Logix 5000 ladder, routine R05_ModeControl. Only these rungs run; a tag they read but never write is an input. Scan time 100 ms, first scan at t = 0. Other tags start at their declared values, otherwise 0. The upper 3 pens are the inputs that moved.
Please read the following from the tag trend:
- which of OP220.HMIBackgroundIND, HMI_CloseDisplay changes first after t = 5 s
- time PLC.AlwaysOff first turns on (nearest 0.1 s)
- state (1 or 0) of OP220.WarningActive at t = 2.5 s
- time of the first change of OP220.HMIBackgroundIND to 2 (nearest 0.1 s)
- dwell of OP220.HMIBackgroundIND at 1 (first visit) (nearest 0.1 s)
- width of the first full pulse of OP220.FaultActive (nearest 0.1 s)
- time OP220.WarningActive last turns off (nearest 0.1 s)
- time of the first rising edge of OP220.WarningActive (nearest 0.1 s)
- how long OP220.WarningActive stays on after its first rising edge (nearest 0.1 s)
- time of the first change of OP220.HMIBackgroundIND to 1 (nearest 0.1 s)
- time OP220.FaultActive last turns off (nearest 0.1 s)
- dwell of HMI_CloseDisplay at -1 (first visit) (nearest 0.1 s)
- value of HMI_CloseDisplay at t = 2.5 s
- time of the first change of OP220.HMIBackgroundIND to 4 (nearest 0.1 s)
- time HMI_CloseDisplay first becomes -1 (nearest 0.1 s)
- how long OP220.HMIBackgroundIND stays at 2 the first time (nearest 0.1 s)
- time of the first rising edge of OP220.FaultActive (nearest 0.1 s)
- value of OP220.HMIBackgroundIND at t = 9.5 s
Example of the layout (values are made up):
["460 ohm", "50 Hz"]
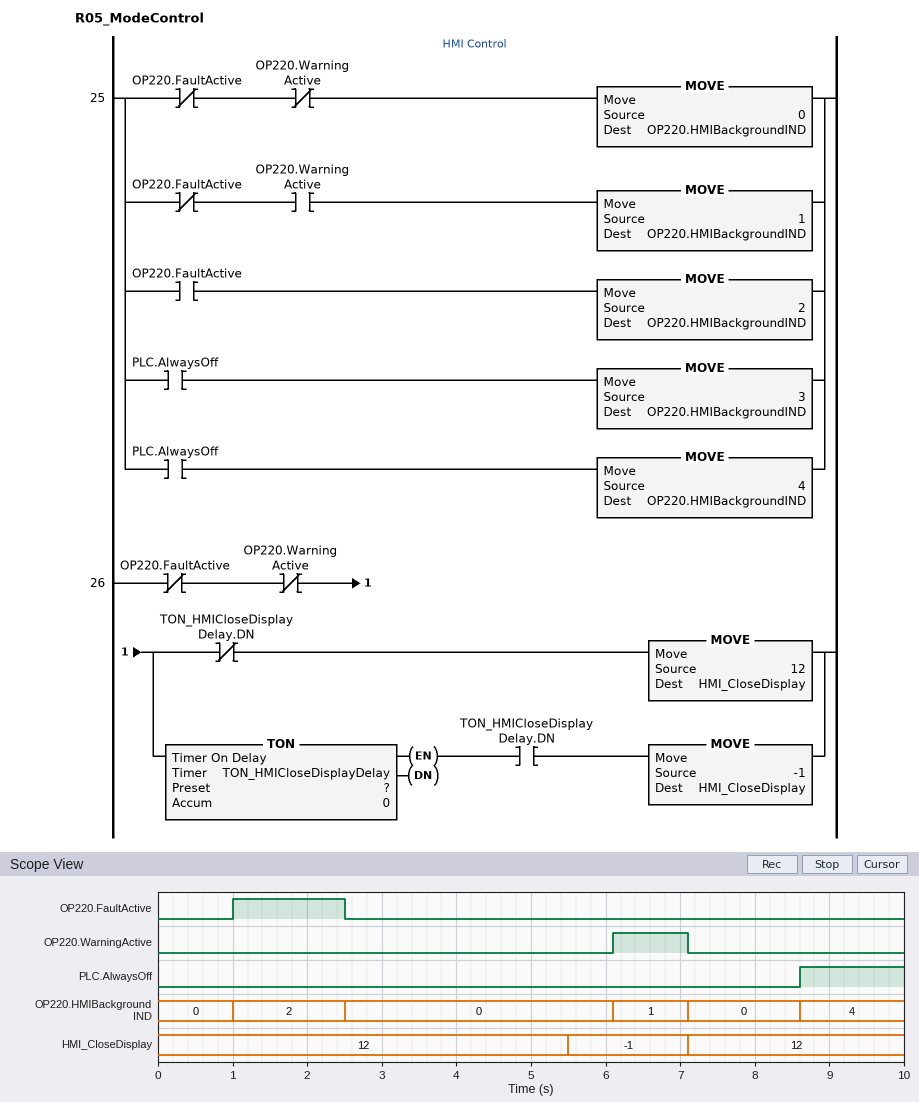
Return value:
["HMI_CloseDisplay", "8.6 s", "0", "1.0 s", "1.0 s", "1.5 s", "7.1 s", "6.1 s", "1.0 s", "6.1 s", "2.5 s", "1.6 s", "12", "8.6 s", "5.5 s", "1.5 s", "1.0 s", "4"]
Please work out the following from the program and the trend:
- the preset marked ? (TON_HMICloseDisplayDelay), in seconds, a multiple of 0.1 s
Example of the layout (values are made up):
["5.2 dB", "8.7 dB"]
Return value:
["3.0 s"]
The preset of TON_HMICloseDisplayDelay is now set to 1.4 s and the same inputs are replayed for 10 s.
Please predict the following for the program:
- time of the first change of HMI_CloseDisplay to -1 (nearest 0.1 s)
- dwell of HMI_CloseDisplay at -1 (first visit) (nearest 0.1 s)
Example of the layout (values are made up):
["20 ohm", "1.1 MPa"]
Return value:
["3.9 s", "3.2 s"]
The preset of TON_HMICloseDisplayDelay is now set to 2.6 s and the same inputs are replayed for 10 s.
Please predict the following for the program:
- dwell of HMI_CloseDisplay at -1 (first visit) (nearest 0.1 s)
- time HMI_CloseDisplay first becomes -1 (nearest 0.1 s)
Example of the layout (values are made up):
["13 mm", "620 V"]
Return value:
["2.0 s", "5.1 s"]
